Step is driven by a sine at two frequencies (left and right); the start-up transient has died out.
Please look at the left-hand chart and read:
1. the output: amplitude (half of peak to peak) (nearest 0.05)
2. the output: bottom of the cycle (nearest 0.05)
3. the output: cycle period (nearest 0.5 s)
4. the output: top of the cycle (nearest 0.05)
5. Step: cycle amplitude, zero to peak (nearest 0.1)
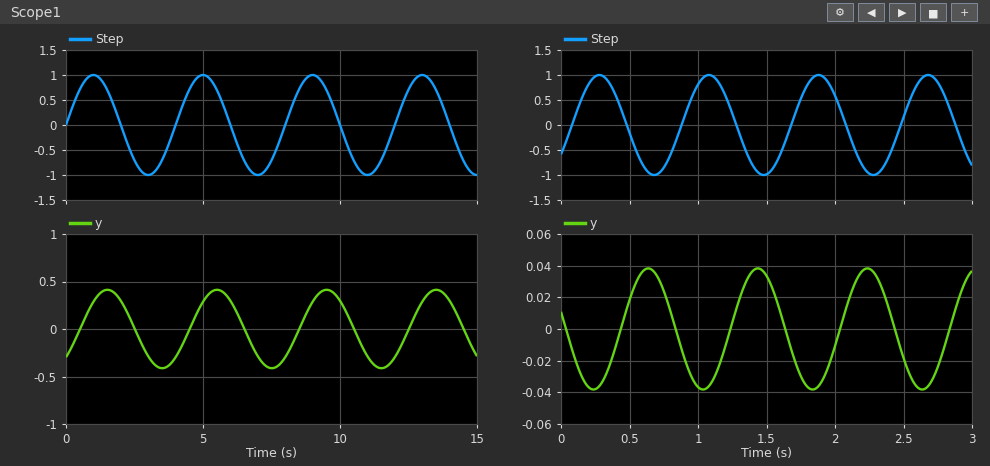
0.40
-0.40
4.0 s
0.40
1.0
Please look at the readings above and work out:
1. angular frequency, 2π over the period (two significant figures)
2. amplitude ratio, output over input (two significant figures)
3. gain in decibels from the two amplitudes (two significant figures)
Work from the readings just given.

1.6 rad/s
0.40
-8.0 dB
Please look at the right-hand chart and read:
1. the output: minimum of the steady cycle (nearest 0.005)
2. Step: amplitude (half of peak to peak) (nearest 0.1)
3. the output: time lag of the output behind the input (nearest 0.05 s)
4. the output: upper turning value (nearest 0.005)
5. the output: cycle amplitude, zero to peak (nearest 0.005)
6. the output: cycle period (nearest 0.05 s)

-0.040
1.0
0.35 s
0.040
0.040
0.80 s
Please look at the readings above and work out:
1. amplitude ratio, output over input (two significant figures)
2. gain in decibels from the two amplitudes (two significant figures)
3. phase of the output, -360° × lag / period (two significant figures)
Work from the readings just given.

0.040
-28 dB
-160°
